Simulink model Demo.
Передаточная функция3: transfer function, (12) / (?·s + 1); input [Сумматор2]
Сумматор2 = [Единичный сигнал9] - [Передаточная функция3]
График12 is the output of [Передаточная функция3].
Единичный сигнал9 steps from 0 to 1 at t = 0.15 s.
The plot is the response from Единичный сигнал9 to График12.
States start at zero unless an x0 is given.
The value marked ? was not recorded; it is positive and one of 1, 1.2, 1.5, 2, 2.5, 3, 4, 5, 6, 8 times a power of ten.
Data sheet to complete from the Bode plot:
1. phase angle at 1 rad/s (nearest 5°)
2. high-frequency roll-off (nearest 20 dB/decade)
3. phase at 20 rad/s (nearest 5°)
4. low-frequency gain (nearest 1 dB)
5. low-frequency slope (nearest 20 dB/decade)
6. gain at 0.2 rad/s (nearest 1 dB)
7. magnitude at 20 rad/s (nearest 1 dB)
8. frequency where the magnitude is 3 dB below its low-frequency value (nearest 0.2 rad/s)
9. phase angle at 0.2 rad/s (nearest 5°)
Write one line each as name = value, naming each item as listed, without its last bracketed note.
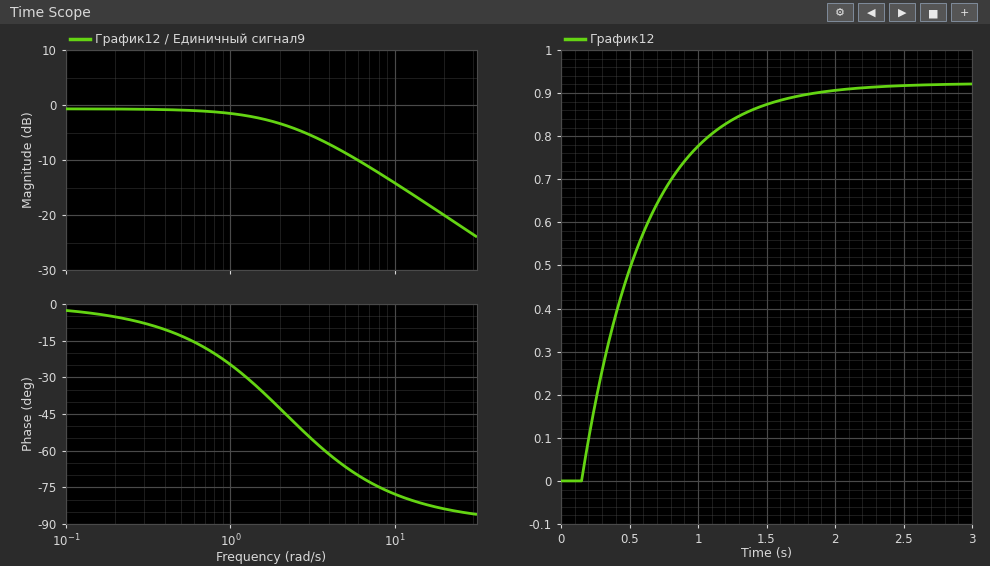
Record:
phase angle at 1 rad/s = -25°
high-frequency roll-off = -20 dB/decade
phase at 20 rad/s = -85°
low-frequency gain = -1 dB
low-frequency slope = 0 dB/decade
gain at 0.2 rad/s = -1 dB
magnitude at 20 rad/s = -20 dB
frequency where the magnitude is 3 dB below its low-frequency value = 2.2 rad/s
phase angle at 0.2 rad/s = -5°
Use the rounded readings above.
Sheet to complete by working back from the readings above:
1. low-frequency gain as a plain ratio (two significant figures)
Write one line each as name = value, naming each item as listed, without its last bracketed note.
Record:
low-frequency gain as a plain ratio = 0.89
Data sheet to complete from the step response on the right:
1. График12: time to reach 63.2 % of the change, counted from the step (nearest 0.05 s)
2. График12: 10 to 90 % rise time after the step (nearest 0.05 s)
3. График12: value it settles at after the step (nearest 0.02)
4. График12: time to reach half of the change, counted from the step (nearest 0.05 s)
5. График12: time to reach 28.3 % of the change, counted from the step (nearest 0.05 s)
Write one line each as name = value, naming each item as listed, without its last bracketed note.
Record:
График12: time to reach 63.2 % of the change, counted from the step = 0.45 s
График12: 10 to 90 % rise time after the step = 1.00 s
График12: value it settles at after the step = 0.92
График12: time to reach half of the change, counted from the step = 0.30 s
График12: time to reach 28.3 % of the change, counted from the step = 0.15 s
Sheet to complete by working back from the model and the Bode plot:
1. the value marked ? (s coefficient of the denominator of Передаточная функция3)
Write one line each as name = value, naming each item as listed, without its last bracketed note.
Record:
the value marked ? = 6
